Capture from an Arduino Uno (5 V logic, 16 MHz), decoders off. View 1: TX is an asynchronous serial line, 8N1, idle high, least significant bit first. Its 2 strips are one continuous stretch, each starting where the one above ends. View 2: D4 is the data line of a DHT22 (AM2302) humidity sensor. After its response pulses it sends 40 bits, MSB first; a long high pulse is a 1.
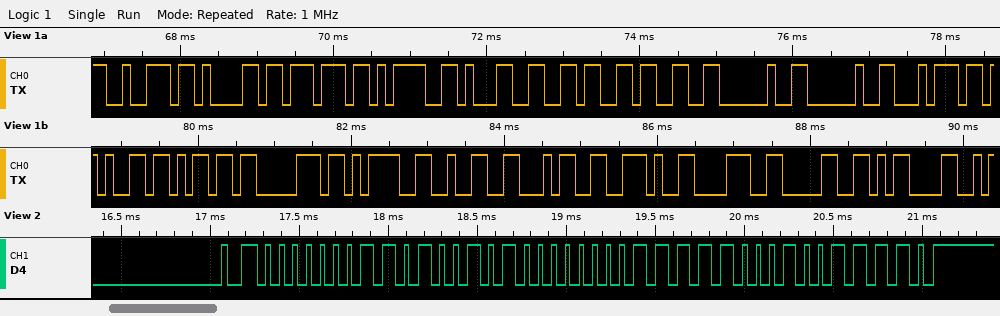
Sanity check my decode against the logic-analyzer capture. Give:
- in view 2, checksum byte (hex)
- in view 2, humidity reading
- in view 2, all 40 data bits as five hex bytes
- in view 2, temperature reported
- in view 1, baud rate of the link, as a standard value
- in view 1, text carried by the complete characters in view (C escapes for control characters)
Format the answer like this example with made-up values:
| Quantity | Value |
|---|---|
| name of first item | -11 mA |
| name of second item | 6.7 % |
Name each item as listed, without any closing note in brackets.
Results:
| Quantity | Value |
|---|---|
| in view 2, checksum byte | 0x9E |
| in view 2, humidity reading | 42.1 % |
| in view 2, all 40 data bits as five hex bytes | 01 A5 00 F8 9E |
| in view 2, temperature reported | 24.8 °C |
| in view 1, baud rate of the link, as a standard value | 9600 baud |
| in view 1, text carried by the complete characters in view | "raw=163  temp=24.80\r" |
